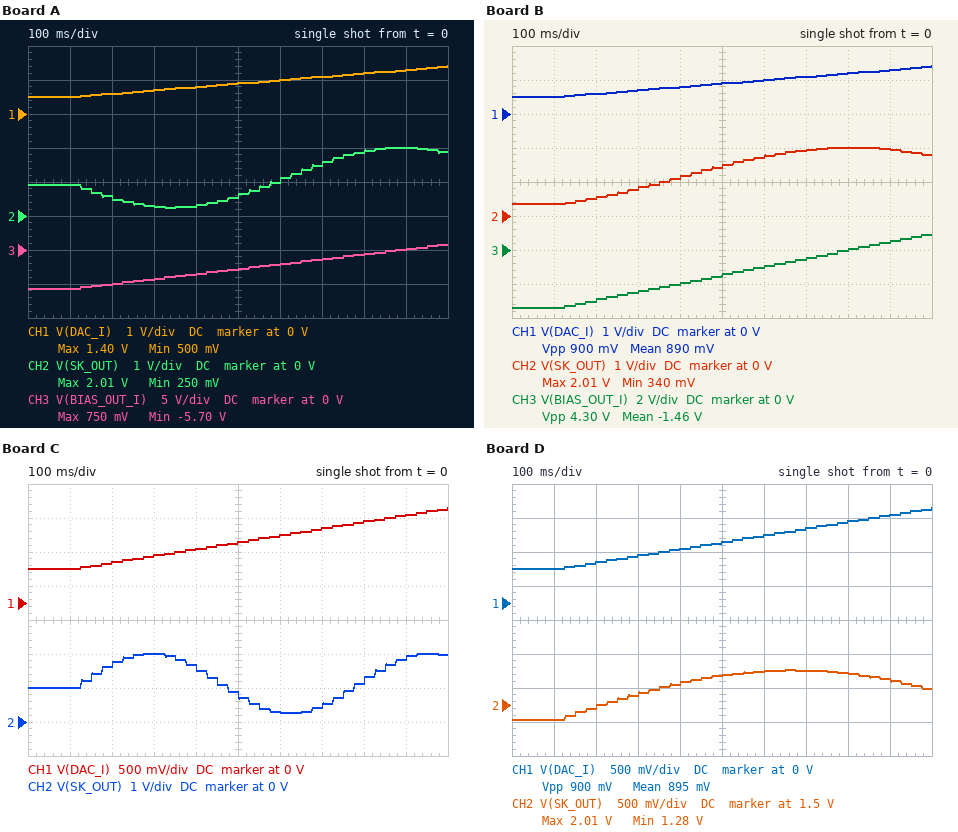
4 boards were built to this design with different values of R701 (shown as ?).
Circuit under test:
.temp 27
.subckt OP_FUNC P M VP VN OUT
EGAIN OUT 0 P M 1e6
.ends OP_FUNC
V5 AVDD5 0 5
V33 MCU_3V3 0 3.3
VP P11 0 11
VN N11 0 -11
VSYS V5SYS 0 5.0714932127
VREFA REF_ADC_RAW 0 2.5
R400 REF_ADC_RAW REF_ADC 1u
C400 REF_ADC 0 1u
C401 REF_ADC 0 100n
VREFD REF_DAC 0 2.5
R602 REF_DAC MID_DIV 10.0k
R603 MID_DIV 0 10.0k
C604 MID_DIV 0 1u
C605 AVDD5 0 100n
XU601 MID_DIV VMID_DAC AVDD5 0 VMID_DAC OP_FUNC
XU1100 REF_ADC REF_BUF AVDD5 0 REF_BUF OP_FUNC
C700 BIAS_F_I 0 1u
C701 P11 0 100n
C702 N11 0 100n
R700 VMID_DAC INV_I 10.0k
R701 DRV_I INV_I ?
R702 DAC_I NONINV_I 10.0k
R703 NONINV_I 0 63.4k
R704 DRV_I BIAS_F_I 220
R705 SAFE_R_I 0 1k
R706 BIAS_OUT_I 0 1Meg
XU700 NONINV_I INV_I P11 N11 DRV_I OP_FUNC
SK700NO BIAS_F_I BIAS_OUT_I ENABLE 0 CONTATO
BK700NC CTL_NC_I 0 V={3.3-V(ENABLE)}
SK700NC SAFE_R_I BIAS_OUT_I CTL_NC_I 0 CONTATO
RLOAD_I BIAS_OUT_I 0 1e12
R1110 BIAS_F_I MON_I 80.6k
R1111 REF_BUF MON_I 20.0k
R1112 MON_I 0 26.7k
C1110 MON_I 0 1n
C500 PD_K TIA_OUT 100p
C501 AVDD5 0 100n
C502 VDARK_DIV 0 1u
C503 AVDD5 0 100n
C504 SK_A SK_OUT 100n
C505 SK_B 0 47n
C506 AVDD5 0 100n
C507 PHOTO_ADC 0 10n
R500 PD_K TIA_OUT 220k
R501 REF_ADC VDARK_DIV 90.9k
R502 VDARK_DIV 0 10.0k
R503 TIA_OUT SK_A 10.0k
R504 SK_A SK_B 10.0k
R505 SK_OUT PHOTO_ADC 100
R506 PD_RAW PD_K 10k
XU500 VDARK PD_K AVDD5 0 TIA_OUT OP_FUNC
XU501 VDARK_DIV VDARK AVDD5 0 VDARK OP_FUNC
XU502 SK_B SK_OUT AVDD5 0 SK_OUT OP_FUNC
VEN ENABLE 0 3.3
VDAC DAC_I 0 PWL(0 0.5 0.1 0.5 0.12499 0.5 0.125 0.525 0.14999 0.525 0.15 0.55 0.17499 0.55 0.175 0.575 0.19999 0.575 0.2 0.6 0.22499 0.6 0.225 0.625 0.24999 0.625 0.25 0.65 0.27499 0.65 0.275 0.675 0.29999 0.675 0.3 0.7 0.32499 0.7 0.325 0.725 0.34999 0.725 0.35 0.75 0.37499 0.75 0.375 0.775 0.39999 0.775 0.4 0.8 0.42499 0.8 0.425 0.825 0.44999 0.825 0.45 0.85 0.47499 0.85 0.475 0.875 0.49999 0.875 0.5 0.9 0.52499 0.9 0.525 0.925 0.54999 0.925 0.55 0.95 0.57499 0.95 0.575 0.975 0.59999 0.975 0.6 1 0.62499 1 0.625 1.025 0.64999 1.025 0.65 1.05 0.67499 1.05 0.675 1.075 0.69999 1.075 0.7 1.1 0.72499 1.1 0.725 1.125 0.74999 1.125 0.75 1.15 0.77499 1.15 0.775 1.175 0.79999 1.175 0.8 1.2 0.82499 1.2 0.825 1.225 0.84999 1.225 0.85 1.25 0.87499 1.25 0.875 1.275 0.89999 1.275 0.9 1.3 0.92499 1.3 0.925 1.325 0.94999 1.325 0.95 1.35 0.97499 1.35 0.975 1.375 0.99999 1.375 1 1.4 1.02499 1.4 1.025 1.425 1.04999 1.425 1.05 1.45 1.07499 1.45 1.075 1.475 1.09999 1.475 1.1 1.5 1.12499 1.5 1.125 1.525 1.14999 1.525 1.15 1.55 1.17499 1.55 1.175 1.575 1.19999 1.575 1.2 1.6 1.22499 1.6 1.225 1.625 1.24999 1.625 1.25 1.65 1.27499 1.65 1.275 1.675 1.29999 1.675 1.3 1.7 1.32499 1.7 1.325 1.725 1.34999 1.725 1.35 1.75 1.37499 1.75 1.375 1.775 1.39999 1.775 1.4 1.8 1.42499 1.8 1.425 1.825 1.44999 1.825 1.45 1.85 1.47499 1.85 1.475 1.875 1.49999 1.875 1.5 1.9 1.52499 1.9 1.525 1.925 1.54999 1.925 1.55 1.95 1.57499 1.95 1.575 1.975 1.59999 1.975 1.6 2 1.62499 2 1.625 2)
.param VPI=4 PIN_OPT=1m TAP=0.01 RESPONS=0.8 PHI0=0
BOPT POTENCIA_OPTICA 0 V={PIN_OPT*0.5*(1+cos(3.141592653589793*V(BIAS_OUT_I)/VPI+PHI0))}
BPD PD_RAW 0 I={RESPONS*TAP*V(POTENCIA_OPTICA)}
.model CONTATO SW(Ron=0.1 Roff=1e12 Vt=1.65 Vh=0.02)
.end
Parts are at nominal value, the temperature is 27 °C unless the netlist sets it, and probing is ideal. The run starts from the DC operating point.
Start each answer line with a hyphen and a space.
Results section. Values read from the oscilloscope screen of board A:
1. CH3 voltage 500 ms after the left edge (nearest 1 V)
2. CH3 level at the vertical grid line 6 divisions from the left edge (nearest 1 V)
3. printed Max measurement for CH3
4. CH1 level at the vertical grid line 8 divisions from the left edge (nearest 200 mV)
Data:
- -3 V
- -2 V
- 750 mV
- 1.2 V
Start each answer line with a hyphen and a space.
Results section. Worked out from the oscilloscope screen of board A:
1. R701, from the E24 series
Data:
- 75 kΩ
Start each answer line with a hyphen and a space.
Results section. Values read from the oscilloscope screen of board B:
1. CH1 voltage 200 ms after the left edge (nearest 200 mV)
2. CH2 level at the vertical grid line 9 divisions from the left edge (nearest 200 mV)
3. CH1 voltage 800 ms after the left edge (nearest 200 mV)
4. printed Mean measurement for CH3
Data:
- 600 mV
- 2.0 V
- 1.2 V
- -1.46 V
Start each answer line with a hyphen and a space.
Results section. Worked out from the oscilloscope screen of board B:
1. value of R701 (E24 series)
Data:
- 47 kΩ
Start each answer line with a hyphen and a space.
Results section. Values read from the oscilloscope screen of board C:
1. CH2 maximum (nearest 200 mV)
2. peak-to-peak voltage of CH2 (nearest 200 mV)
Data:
- 2.0 V
- 1.8 V
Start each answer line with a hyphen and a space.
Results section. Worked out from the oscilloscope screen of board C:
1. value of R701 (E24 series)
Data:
- 130 kΩ
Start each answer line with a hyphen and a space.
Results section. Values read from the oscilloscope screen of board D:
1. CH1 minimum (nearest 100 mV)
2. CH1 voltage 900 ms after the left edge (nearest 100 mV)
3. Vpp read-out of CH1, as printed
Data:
- 500 mV
- 1.3 V
- 900 mV
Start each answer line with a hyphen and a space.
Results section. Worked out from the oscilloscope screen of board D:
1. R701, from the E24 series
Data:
- 27 kΩ
